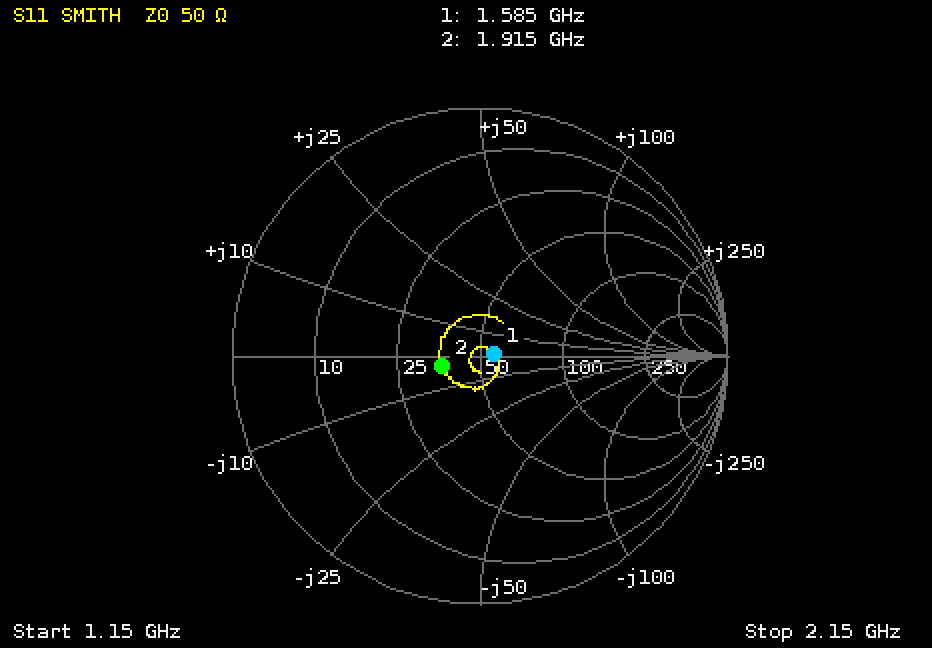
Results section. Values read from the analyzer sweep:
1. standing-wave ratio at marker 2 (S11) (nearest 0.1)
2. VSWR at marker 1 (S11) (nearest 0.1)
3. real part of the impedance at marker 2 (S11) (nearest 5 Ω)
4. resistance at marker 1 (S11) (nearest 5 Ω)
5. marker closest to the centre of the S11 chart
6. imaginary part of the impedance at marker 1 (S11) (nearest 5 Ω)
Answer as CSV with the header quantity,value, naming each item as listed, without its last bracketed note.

quantity,value
standing-wave ratio at marker 2 (S11),1.4
VSWR at marker 1 (S11),1.1
real part of the impedance at marker 2 (S11),35 Ω
resistance at marker 1 (S11),55 Ω
marker closest to the centre of the S11 chart,marker 1
imaginary part of the impedance at marker 1 (S11),0 Ω
